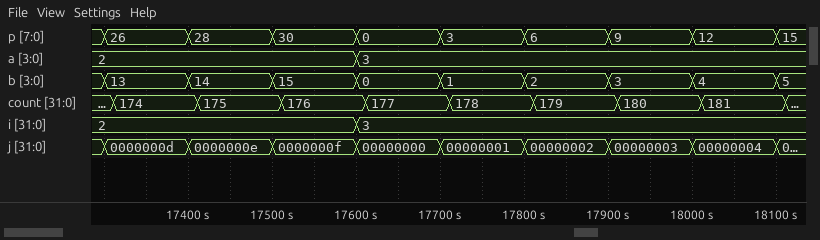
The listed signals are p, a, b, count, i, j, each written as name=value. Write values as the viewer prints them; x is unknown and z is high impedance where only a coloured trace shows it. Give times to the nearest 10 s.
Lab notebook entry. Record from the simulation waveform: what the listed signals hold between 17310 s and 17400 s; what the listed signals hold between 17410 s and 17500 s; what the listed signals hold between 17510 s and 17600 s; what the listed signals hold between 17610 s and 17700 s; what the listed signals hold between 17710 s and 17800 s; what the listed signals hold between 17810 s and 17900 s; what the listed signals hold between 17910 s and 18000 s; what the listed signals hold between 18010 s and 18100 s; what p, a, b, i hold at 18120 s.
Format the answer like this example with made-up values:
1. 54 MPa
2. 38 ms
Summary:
1. p=26, a=2, b=13, count=174, i=2, j=0000000d
2. p=28, a=2, b=14, count=175, i=2, j=0000000e
3. p=30, a=2, b=15, count=176, i=2, j=0000000f
4. p=0, a=3, b=0, count=177, i=3, j=00000000
5. p=3, a=3, b=1, count=178, i=3, j=00000001
6. p=6, a=3, b=2, count=179, i=3, j=00000002
7. p=9, a=3, b=3, count=180, i=3, j=00000003
8. p=12, a=3, b=4, count=181, i=3, j=00000004
9. p=15, a=3, b=5, i=3
